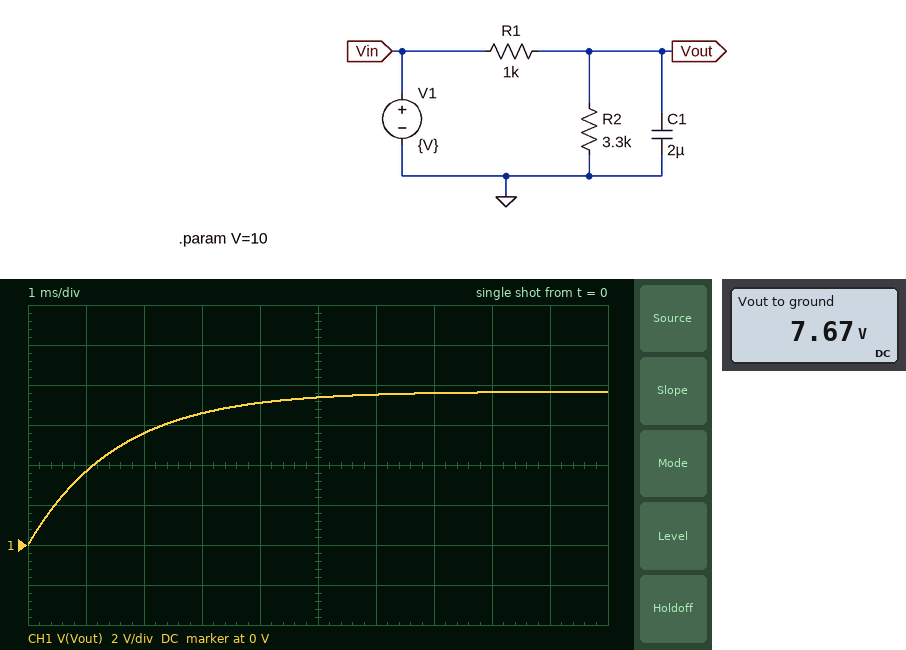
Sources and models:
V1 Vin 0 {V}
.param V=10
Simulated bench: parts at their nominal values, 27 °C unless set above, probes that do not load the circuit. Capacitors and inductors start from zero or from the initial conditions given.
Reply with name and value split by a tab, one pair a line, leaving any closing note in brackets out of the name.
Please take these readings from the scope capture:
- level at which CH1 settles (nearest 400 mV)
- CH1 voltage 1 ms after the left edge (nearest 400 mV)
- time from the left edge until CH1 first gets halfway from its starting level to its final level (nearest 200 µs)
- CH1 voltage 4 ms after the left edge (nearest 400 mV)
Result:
level at which CH1 settles	7.6 V
CH1 voltage 1 ms after the left edge	3.6 V
time from the left edge until CH1 first gets halfway from its starting level to its final level	1.0 ms
CH1 voltage 4 ms after the left edge	7.2 V
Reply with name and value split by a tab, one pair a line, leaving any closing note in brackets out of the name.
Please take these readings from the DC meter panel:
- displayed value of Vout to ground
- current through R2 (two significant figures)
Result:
displayed value of Vout to ground	7.67 V
current through R2	2.3 mA
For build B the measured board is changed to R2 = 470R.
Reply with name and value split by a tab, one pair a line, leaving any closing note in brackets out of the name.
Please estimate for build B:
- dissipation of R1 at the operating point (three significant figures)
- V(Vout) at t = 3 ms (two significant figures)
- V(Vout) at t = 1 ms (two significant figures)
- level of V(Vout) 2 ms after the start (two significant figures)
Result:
dissipation of R1 at the operating point	46.3 mW
V(Vout) at t = 3 ms	3.2 V
V(Vout) at t = 1 ms	2.5 V
level of V(Vout) 2 ms after the start	3.1 V
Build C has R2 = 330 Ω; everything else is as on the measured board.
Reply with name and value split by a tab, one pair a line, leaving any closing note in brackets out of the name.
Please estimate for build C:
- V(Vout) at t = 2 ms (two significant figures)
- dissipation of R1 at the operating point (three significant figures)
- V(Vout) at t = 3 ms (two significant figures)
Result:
V(Vout) at t = 2 ms	2.4 V
dissipation of R1 at the operating point	56.5 mW
V(Vout) at t = 3 ms	2.5 V
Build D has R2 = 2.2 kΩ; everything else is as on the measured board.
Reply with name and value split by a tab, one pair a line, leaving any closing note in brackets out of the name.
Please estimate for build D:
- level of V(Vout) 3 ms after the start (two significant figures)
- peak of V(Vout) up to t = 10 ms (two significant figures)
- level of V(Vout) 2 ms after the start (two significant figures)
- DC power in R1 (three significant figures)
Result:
level of V(Vout) 3 ms after the start	6.1 V
peak of V(Vout) up to t = 10 ms	6.9 V
level of V(Vout) 2 ms after the start	5.3 V
DC power in R1	9.77 mW
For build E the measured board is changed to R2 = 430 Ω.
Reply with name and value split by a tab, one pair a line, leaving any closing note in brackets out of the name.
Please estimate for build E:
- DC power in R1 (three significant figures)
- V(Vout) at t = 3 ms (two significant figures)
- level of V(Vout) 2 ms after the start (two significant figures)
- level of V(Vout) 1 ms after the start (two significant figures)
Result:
DC power in R1	48.9 mW
V(Vout) at t = 3 ms	3.0 V
level of V(Vout) 2 ms after the start	2.9 V
level of V(Vout) 1 ms after the start	2.4 V
